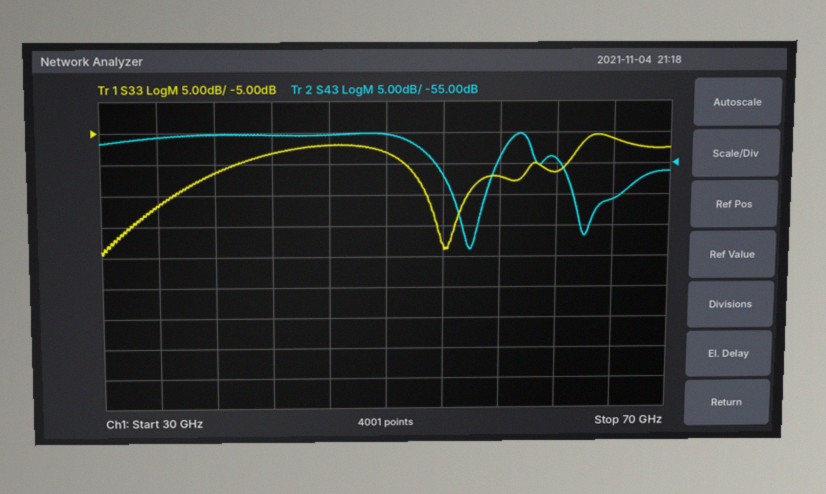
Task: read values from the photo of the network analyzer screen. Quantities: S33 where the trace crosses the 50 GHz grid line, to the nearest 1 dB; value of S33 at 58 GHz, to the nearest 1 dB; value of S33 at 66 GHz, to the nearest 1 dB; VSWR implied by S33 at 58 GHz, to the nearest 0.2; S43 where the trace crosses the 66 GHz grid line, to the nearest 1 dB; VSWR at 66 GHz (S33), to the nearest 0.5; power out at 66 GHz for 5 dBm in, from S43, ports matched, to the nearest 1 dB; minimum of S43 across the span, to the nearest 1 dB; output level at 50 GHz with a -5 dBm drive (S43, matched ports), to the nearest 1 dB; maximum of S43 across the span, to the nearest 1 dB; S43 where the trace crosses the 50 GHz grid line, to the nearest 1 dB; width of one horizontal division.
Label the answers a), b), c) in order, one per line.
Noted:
a) -8 dB
b) -12 dB
c) -6 dB
d) 1.6
e) -61 dB
f) 3.0
g) -56 dBm
h) -69 dB
i) -55 dBm
j) -50 dB
k) -50 dB
l) 4 GHz
